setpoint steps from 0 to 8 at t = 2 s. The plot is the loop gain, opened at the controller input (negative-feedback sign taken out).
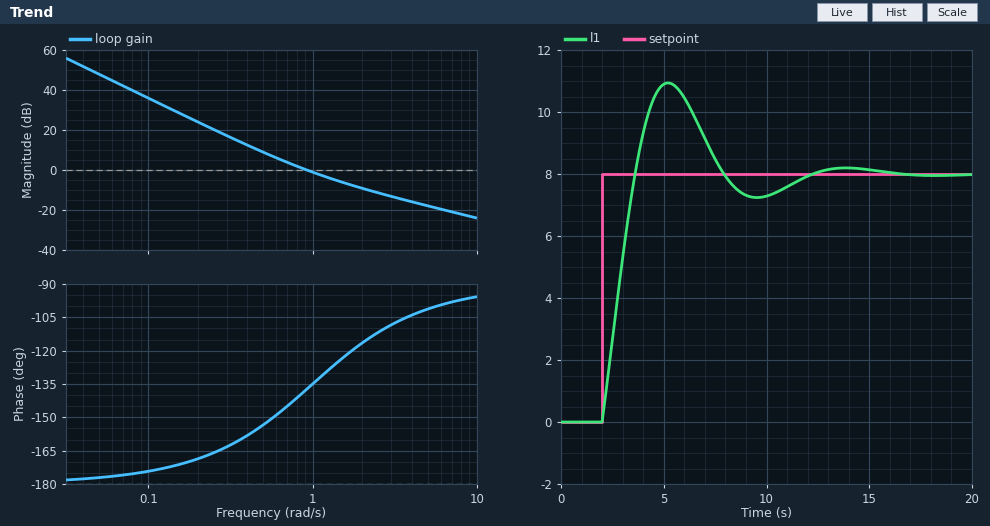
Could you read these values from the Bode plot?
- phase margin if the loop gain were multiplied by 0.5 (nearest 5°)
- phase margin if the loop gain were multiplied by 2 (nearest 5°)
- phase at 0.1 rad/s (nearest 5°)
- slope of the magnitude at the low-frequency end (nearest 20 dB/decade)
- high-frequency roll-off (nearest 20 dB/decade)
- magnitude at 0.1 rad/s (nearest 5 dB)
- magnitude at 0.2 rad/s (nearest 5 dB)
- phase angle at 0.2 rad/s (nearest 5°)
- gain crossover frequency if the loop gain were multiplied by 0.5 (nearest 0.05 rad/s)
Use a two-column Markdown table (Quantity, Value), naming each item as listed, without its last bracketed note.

| Quantity | Value |
|---|---|
| phase margin if the loop gain were multiplied by 0.5 | 30° |
| phase margin if the loop gain were multiplied by 2 | 55° |
| phase at 0.1 rad/s | -175° |
| slope of the magnitude at the low-frequency end | -40 dB/decade |
| high-frequency roll-off | -20 dB/decade |
| magnitude at 0.1 rad/s | 35 dB |
| magnitude at 0.2 rad/s | 25 dB |
| phase angle at 0.2 rad/s | -170° |
| gain crossover frequency if the loop gain were multiplied by 0.5 | 0.60 rad/s |
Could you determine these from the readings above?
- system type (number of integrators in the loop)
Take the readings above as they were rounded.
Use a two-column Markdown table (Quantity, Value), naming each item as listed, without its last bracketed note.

| Quantity | Value |
|---|---|
| system type | 2 |
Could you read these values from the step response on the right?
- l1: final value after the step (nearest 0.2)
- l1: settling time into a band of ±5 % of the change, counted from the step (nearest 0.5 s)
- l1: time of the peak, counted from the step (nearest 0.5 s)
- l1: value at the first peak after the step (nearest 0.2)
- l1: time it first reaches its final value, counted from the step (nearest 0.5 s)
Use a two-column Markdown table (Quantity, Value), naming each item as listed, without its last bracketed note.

| Quantity | Value |
|---|---|
| l1: final value after the step | 8.0 |
| l1: settling time into a band of ±5 % of the change, counted from the step | 9.0 s |
| l1: time of the peak, counted from the step | 3.0 s |
| l1: value at the first peak after the step | 11.0 |
| l1: time it first reaches its final value, counted from the step | 1.5 s |
